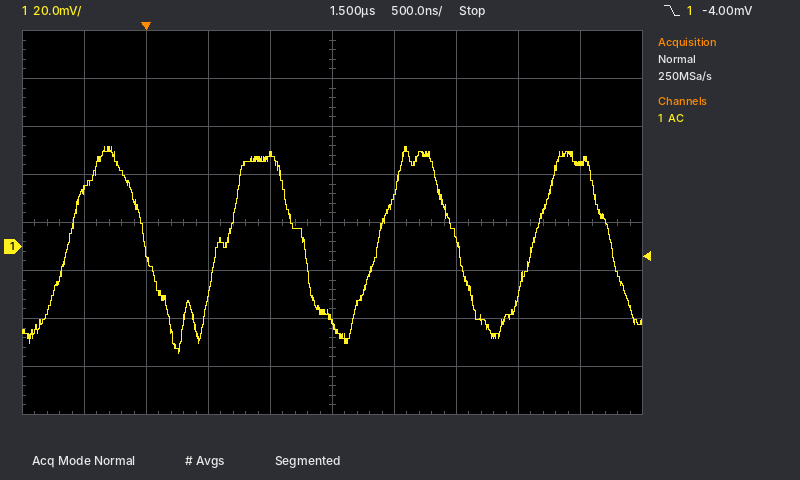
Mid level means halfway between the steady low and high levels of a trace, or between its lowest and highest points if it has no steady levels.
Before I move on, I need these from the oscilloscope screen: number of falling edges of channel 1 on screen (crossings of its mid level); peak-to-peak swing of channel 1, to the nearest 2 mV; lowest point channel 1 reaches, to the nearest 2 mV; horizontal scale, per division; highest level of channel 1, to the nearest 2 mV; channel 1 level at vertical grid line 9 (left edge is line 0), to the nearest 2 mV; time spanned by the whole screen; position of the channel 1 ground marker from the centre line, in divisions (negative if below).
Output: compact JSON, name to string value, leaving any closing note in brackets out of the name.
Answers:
{"number of falling edges of channel 1 on screen": "4", "peak-to-peak swing of channel 1, to the nearest 2 mV": "86 mV", "lowest point channel 1 reaches, to the nearest 2 mV": "-44 mV", "horizontal scale, per division": "500 ns", "highest level of channel 1, to the nearest 2 mV": "42 mV", "channel 1 level at vertical grid line 9 (left edge is line 0), to the nearest 2 mV": "34 mV", "time spanned by the whole screen": "5 µs", "position of the channel 1 ground marker from the centre line, in divisions": "-0.5 div"}
